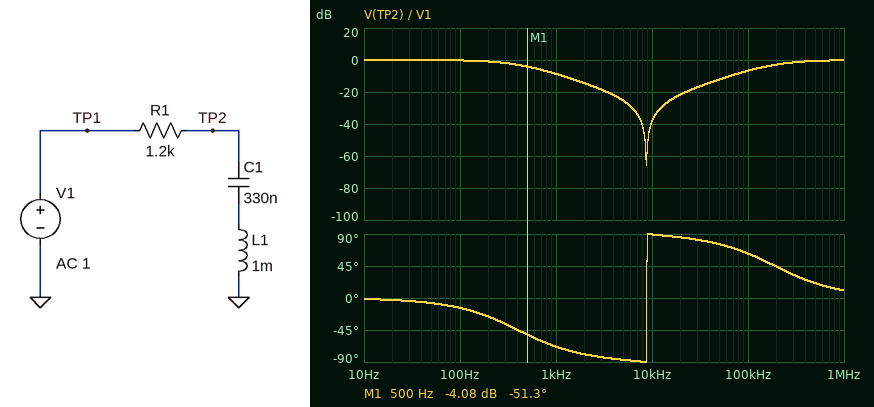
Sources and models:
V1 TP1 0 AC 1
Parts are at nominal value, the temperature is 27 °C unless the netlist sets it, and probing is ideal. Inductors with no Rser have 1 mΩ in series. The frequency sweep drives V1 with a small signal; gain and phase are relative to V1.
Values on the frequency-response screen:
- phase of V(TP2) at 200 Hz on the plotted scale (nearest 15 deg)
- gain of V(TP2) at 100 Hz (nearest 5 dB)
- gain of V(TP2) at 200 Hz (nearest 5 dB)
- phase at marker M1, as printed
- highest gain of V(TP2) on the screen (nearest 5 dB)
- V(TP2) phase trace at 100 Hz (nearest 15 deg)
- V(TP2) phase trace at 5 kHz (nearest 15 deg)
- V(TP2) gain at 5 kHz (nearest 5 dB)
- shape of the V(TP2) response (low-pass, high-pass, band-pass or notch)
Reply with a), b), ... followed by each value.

a) -30 deg
b) 0 dB
c) 0 dB
d) -51.3 deg
e) 0 dB
f) -15 deg
g) -90 deg
h) -25 dB
i) notch
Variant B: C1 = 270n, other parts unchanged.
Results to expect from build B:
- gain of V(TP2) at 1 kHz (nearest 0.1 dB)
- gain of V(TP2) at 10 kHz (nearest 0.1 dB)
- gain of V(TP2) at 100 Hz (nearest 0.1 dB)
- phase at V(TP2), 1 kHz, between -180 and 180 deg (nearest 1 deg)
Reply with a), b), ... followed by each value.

a) -7.2 dB
b) -49.8 dB
c) -0.2 dB
d) -64 deg
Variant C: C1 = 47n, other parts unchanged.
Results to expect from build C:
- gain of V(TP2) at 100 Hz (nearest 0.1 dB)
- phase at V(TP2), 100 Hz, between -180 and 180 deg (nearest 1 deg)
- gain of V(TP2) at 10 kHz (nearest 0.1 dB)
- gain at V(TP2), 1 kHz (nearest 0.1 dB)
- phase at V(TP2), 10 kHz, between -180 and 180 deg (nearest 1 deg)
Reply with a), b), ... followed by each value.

a) 0 dB
b) -2 deg
c) -13.0 dB
d) -0.5 dB
e) -77 deg
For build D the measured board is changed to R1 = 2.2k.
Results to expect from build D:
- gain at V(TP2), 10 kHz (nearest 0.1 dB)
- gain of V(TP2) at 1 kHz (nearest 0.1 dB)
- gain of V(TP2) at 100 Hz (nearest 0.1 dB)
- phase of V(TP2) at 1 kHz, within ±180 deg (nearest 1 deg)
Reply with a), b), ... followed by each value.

a) -43.6 dB
b) -13.5 dB
c) -0.8 dB
d) -78 deg
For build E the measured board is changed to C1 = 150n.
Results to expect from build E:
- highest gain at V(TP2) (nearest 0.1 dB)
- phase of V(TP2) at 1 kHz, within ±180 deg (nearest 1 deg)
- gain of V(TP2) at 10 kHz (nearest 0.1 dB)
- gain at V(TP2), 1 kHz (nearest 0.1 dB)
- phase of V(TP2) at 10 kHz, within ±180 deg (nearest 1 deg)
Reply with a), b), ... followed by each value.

a) 0 dB
b) -49 deg
c) -28.9 dB
d) -3.6 dB
e) -88 deg
